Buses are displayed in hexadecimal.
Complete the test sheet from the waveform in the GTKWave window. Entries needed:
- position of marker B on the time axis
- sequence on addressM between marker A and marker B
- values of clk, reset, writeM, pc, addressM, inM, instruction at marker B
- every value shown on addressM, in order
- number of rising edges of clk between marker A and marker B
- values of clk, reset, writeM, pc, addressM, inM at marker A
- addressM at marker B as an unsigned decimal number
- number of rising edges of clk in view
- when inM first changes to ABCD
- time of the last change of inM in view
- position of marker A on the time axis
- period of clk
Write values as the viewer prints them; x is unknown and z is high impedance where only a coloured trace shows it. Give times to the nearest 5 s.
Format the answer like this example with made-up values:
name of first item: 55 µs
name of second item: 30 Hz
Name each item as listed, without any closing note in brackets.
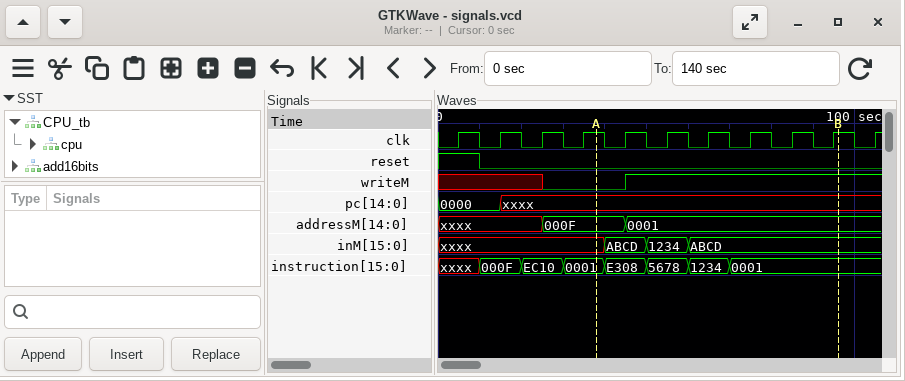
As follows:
position of marker B on the time axis: 95 s
sequence on addressM between marker A and marker B: 000F, 0001
values of clk, reset, writeM, pc, addressM, inM, instruction at marker B: clk=1, reset=0, writeM=1, pc=xxxx, addressM=0001, inM=ABCD, instruction=0001
every value shown on addressM, in order: xxxx, 000F, 0001
number of rising edges of clk between marker A and marker B: 6
values of clk, reset, writeM, pc, addressM, inM at marker A: clk=1, reset=0, writeM=0, pc=xxxx, addressM=000F, inM=xxxx
addressM at marker B as an unsigned decimal number: 1
number of rising edges of clk in view: 11
when inM first changes to ABCD: 40 s
time of the last change of inM in view: 60 s
position of marker A on the time axis: 40 s
period of clk: 10 s
